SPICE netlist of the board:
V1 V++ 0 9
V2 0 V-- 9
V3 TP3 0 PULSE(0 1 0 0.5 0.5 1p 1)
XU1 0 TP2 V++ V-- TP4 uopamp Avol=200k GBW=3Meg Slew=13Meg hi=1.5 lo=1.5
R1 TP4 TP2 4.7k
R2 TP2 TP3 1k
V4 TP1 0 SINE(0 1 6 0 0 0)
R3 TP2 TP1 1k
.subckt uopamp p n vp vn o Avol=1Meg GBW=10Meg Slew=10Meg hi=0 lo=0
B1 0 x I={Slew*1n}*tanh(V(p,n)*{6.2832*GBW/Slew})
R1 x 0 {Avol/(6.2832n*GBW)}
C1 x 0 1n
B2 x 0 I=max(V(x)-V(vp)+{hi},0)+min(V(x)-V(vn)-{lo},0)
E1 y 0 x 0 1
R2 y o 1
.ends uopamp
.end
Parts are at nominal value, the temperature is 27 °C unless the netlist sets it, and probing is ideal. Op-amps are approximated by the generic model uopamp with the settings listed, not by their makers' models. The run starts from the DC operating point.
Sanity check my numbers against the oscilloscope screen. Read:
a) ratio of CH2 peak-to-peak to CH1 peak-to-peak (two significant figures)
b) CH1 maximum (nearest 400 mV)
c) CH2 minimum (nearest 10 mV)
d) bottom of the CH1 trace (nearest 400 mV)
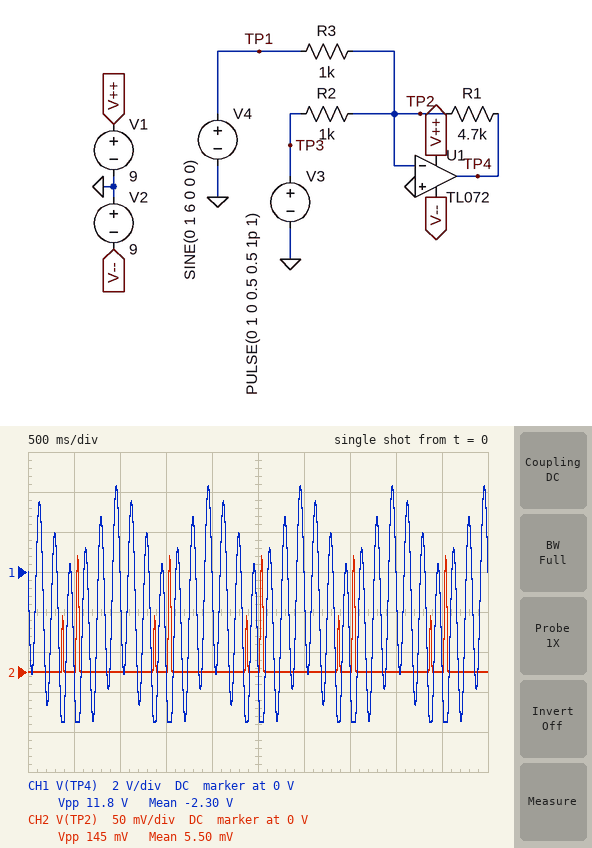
0.012
4.4 V
0 V
-7.6 V
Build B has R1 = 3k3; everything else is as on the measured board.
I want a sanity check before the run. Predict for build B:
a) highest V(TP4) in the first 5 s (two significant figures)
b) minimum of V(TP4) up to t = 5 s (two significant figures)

3.0 V
-6.3 V
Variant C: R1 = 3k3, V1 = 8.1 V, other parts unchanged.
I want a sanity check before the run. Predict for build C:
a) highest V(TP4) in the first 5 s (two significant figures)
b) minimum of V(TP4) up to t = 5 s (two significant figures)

3.0 V
-6.3 V
